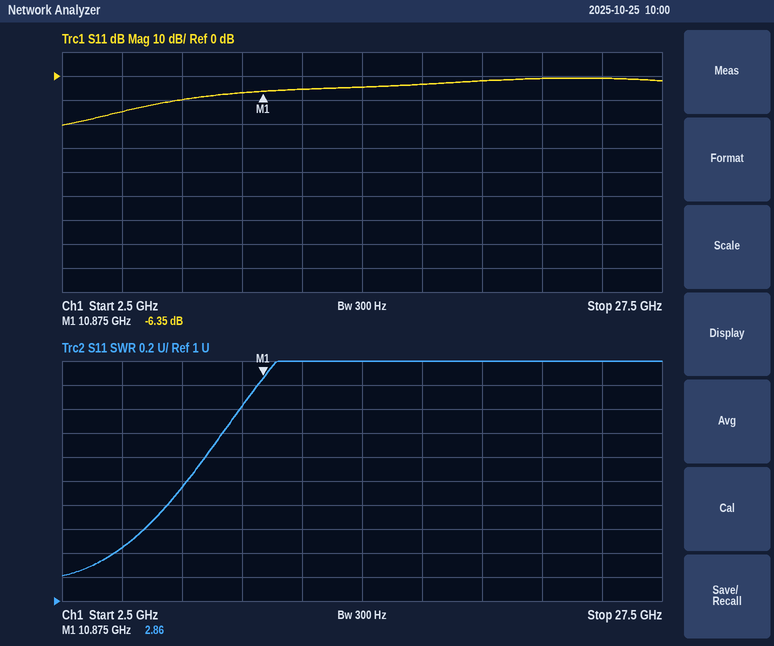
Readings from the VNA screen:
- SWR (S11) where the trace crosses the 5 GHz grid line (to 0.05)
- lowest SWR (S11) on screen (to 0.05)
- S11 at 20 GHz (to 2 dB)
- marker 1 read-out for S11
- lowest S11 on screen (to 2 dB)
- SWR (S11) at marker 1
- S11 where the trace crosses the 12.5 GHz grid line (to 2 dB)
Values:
1.45
1.20
-2 dB
-6.35 dB
-20 dB
2.86
-6 dB
